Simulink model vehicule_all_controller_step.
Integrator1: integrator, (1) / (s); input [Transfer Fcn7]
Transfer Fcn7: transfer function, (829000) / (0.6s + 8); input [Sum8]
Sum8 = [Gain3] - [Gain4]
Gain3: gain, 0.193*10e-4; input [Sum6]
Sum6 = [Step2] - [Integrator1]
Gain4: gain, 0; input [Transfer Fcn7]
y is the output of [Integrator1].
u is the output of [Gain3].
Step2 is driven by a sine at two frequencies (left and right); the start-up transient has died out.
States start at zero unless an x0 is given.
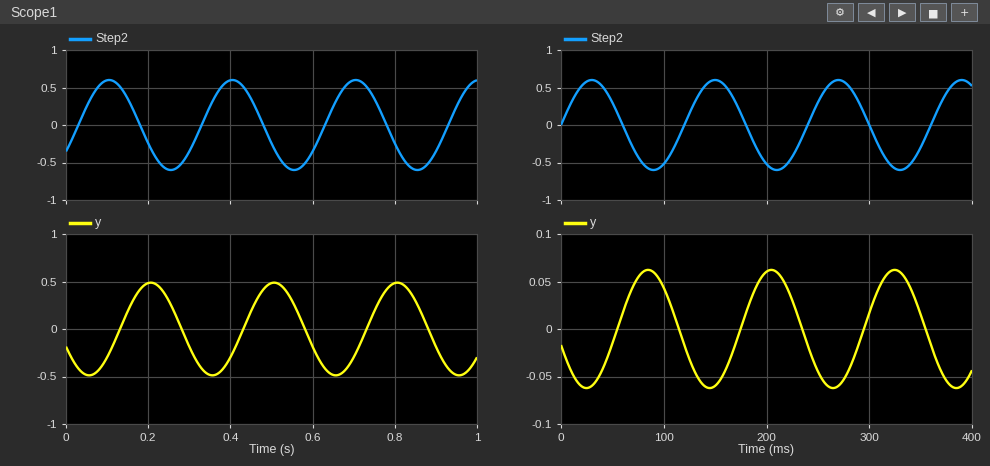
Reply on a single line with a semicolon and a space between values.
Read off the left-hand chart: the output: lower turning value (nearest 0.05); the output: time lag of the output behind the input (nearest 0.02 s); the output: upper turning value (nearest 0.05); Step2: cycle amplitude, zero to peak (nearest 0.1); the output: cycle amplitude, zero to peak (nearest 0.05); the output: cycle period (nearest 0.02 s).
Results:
-0.50; 0.10 s; 0.50; 0.6; 0.50; 0.30 s
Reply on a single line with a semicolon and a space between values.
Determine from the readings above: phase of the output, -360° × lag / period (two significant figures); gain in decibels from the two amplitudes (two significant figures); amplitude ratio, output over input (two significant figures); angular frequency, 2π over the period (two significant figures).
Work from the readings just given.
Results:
-120°; -1.6 dB; 0.83; 21 rad/s
